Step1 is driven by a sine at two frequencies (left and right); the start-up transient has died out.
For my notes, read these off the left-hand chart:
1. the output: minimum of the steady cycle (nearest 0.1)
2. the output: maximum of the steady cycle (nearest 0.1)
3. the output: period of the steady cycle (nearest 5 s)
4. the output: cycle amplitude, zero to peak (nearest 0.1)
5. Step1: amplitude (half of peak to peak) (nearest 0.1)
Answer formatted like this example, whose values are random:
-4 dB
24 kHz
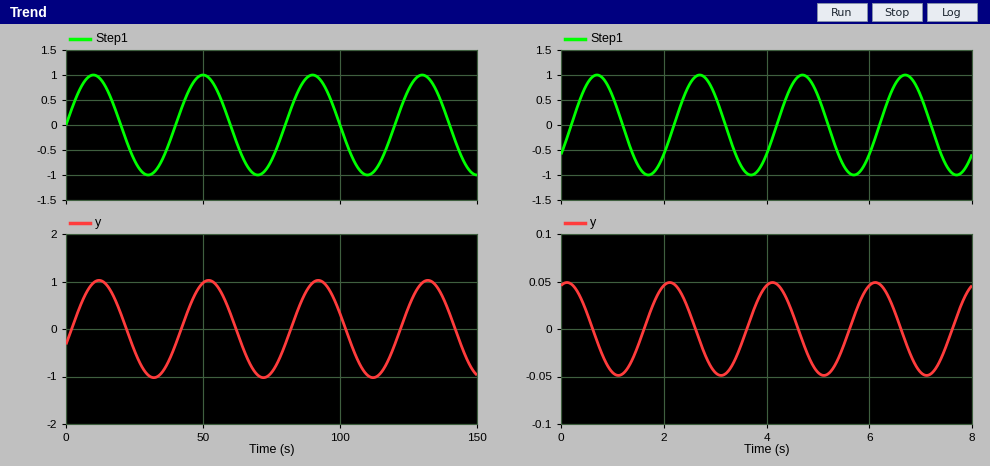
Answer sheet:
-1.0
1.0
40 s
1.0
1.0
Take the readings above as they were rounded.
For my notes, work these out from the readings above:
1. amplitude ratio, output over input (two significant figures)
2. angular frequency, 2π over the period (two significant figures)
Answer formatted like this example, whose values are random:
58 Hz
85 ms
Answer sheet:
1.0
0.16 rad/s
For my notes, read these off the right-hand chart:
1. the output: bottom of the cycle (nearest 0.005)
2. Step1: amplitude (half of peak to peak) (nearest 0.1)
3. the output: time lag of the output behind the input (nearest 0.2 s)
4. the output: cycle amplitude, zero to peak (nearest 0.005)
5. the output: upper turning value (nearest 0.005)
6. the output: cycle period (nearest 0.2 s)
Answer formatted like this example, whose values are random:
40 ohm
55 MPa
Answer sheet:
-0.050
1.0
1.4 s
0.050
0.050
2.0 s
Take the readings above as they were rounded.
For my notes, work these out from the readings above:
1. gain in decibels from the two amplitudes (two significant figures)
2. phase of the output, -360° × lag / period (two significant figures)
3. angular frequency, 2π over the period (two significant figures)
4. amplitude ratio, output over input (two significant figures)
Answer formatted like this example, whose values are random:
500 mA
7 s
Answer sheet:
-26 dB
-250°
3.1 rad/s
0.050
